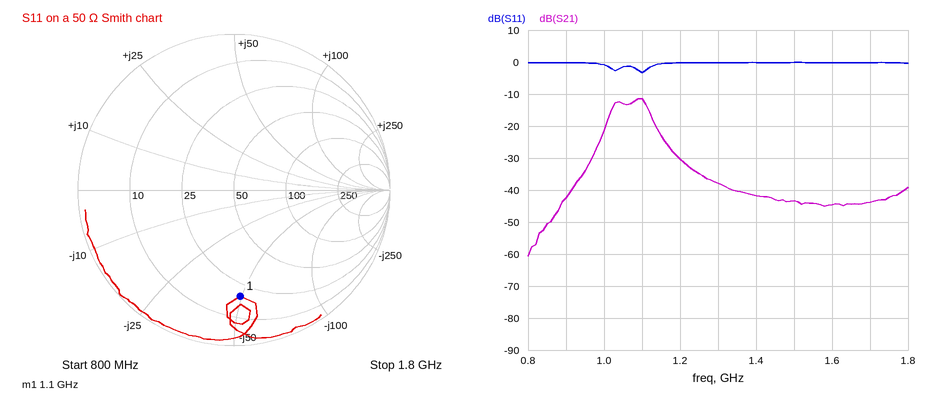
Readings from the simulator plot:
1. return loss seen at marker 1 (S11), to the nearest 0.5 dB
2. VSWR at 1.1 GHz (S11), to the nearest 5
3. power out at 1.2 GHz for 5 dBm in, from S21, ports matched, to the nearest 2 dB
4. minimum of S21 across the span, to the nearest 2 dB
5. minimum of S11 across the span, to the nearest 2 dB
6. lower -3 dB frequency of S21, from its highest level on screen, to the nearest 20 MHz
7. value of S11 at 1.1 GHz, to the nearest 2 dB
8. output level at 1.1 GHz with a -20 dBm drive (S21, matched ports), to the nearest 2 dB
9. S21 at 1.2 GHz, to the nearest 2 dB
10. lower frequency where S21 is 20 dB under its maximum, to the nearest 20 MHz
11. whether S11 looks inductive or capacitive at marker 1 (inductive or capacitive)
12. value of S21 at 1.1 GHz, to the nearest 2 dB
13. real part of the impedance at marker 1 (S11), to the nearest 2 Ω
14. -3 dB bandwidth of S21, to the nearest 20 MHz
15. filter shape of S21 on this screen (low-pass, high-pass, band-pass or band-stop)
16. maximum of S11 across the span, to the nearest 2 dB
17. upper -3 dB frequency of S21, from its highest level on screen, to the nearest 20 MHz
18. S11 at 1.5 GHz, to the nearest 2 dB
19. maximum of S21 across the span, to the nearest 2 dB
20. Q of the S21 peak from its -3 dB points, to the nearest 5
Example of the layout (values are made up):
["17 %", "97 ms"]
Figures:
["3.5 dB", "5", "-26 dBm", "-60 dB", "-4 dB", "1.02 GHz", "-4 dB", "-32 dBm", "-30 dB", "960 MHz", "capacitive", "-12 dB", "20 Ω", "100 MHz", "band-pass", "0 dB", "1.12 GHz", "0 dB", "-12 dB", "10"]
